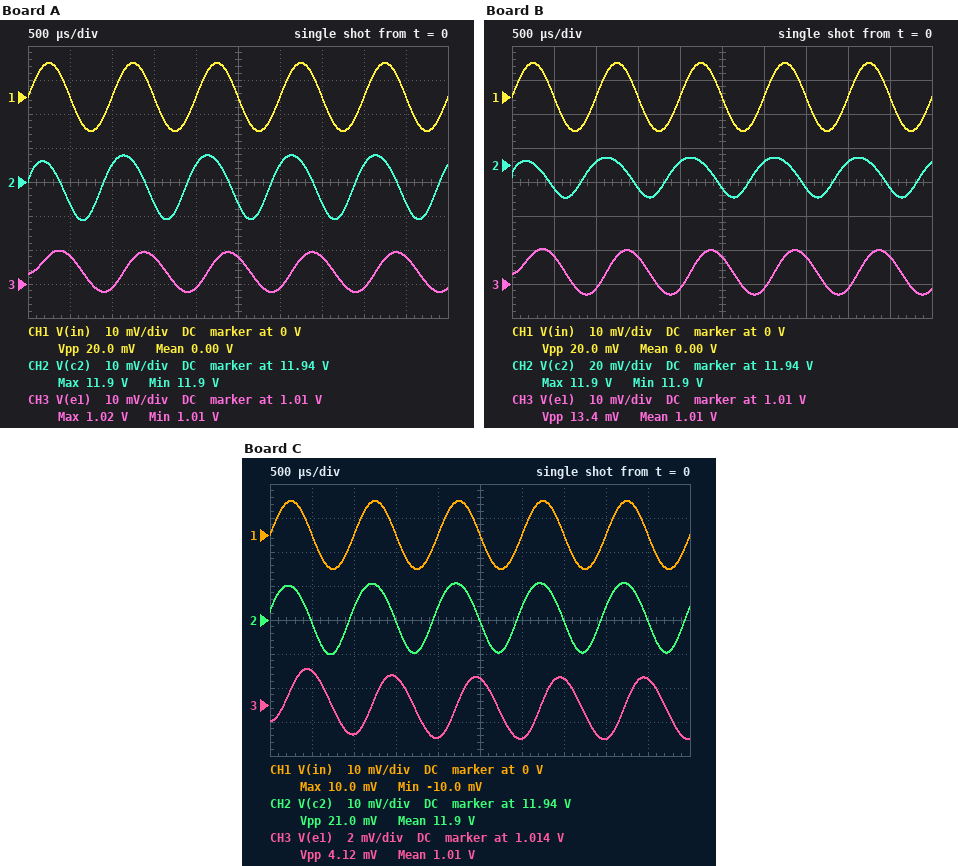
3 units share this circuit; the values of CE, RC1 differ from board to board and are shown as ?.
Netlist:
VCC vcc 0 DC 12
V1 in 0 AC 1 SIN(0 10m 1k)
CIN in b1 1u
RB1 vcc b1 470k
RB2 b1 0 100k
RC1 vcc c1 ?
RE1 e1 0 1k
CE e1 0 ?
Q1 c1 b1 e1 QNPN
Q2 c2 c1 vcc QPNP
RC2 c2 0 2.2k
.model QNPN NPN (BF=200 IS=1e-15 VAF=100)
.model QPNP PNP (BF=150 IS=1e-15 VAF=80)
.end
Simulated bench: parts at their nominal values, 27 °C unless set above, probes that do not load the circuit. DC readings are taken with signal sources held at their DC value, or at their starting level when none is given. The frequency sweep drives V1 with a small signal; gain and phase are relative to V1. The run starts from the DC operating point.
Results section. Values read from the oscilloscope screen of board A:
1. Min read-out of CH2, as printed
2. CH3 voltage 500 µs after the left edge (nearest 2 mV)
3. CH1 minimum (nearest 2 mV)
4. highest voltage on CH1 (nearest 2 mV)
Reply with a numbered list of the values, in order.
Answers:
1. 11.9 V
2. 1.018 V
3. -10 mV
4. 10 mV
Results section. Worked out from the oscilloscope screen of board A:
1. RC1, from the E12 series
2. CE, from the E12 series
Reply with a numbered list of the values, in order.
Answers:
1. 2.7 kΩ
2. 8.2 µF
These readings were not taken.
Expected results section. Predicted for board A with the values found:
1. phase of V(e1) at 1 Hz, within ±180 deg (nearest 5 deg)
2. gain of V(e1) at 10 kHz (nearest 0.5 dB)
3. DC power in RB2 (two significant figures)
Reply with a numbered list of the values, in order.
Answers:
1. 70 deg
2. -22.5 dB
3. 30 µW
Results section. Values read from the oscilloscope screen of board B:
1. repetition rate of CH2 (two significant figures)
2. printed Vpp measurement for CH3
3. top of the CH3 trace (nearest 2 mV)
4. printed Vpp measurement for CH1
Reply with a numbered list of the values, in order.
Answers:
1. 1.0 kHz
2. 13.4 mV
3. 1.020 V
4. 20.0 mV
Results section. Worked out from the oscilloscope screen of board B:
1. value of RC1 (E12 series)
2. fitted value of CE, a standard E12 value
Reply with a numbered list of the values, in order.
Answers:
1. 1.8 kΩ
2. 6.8 µF
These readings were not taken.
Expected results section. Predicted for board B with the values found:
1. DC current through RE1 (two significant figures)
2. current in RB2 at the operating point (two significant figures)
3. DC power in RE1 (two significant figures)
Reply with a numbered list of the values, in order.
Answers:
1. 1.0 mA
2. 17 µA
3. 1.0 mW
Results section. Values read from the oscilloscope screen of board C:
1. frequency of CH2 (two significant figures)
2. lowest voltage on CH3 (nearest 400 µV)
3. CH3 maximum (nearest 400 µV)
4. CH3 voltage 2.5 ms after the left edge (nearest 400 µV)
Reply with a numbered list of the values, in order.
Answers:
1. 1.0 kHz
2. 1.0120 V
3. 1.0160 V
4. 1.0156 V
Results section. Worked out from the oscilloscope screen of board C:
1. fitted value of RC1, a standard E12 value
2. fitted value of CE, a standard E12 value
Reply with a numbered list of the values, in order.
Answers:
1. 3.9 kΩ
2. 33 µF
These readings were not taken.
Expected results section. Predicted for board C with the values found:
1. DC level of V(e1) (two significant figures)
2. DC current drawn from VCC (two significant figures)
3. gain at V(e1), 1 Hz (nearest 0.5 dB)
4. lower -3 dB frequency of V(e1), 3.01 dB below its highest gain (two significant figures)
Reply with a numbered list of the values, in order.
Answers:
1. 1.0 V
2. 6.5 mA
3. -9.5 dB
4. 2.3 Hz
